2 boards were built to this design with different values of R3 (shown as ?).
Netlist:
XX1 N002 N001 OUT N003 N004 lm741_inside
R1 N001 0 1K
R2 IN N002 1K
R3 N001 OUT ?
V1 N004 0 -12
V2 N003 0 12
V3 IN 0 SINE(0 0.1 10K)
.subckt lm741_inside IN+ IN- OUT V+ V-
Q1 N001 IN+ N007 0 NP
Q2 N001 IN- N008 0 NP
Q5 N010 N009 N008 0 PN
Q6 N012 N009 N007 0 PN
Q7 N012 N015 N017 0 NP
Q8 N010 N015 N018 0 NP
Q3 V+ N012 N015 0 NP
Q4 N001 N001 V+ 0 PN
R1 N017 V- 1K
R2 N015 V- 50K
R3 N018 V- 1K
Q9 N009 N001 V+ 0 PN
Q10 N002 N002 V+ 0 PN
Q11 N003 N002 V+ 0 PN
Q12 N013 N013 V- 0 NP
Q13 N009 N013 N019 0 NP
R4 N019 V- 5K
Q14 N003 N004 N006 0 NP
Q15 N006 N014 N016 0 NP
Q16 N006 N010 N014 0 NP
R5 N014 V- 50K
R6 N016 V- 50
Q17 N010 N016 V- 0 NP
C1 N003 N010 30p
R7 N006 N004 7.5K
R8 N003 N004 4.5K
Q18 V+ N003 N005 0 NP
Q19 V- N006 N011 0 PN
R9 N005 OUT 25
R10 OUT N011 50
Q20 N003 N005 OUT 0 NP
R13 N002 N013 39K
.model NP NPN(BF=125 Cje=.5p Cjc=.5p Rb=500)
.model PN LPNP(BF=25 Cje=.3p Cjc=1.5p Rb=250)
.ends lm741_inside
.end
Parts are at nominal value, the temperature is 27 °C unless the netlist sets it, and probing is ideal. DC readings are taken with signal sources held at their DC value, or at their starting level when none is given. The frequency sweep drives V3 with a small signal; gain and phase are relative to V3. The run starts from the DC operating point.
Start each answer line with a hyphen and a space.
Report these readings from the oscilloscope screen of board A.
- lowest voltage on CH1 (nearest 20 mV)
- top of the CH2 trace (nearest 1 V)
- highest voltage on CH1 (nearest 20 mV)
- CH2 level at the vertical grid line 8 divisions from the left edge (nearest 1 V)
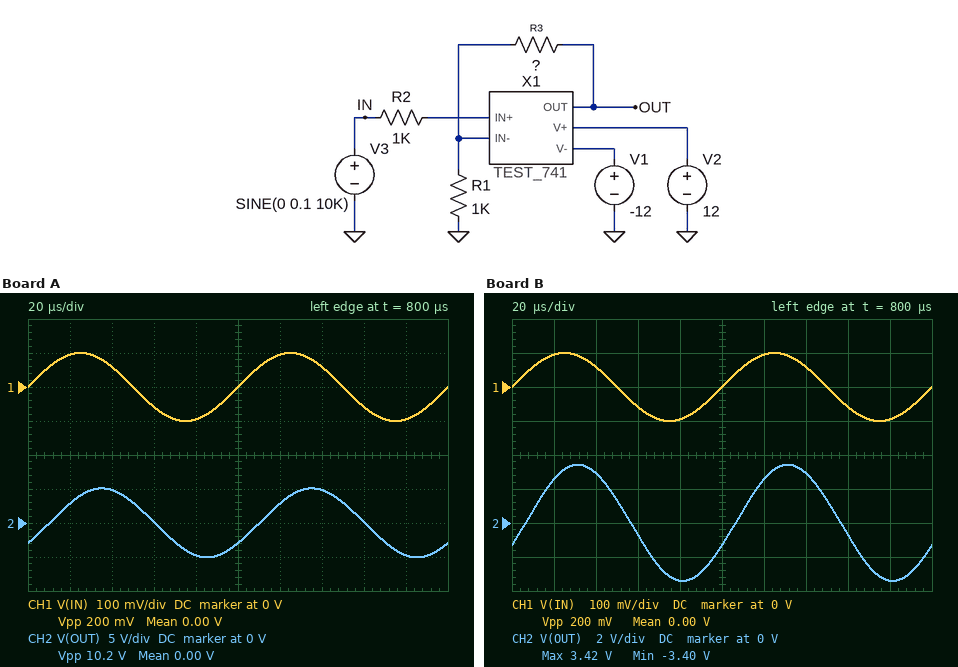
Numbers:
- -100 mV
- 5 V
- 100 mV
- 0 V
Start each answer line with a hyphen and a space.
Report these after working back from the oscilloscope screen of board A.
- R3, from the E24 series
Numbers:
- 62 kΩ
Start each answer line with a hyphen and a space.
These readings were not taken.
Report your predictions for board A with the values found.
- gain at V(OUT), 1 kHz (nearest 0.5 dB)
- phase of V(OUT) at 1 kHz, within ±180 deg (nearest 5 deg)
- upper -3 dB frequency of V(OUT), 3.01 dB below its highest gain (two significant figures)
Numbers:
- 36.0 dB
- -5 deg
- 13 kHz
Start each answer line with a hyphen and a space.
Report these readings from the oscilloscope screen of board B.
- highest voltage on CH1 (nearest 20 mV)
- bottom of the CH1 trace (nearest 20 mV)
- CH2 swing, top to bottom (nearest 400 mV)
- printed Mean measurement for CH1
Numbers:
- 100 mV
- -100 mV
- 6.8 V
- 0.00 V
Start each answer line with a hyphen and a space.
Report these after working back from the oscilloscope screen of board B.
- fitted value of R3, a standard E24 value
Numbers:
- 36 kΩ
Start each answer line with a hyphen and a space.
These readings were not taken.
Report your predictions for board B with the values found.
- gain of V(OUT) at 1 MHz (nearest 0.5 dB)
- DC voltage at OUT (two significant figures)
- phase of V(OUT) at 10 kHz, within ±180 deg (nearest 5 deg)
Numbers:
- -2.0 dB
- 11 mV
- -25 deg
